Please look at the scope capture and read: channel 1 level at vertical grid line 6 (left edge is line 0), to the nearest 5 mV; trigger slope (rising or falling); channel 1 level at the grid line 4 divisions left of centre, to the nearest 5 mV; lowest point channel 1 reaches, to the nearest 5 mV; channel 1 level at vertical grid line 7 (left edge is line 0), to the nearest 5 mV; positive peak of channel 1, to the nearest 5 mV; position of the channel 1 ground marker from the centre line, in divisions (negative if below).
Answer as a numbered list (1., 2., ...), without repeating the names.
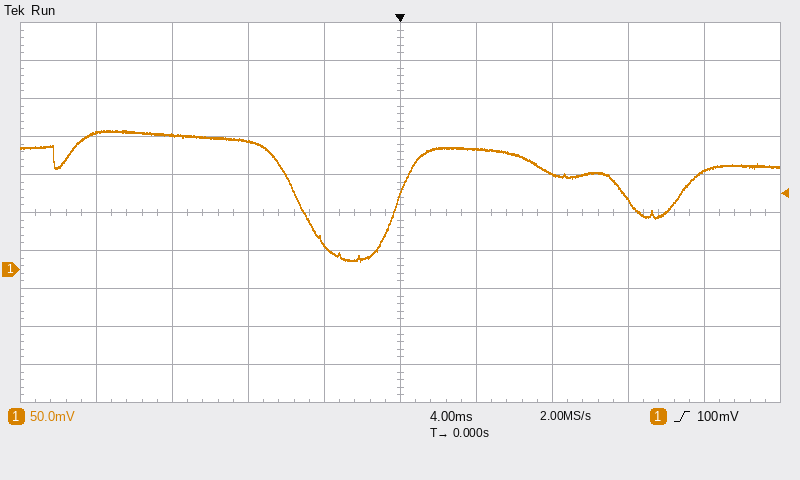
1. 160 mV
2. rising
3. 180 mV
4. 10 mV
5. 125 mV
6. 185 mV
7. -1.5 div
